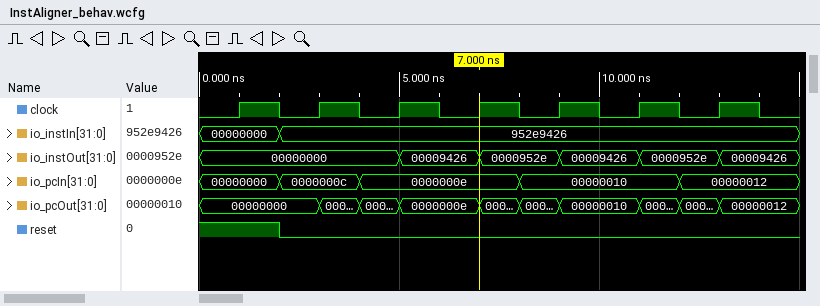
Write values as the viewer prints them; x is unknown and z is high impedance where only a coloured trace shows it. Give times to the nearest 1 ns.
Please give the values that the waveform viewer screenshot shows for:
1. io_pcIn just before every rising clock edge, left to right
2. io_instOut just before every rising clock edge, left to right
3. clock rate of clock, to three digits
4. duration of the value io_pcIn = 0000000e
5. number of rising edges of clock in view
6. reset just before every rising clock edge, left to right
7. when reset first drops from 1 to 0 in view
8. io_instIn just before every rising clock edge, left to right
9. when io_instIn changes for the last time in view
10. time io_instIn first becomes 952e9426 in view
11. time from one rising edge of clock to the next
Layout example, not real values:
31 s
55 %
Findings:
00000000, 0000000c, 0000000e, 0000000e, 00000010, 00000010, 00000012
00000000, 00000000, 00000000, 00009426, 0000952e, 00009426, 0000952e
500 MHz
4 ns
7
1 0 0 0 0 0 0
2 ns
00000000, 952e9426, 952e9426, 952e9426, 952e9426, 952e9426, 952e9426
2 ns
2 ns
2 ns
